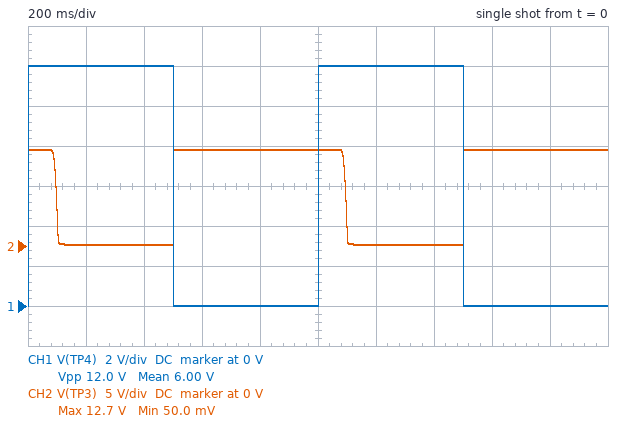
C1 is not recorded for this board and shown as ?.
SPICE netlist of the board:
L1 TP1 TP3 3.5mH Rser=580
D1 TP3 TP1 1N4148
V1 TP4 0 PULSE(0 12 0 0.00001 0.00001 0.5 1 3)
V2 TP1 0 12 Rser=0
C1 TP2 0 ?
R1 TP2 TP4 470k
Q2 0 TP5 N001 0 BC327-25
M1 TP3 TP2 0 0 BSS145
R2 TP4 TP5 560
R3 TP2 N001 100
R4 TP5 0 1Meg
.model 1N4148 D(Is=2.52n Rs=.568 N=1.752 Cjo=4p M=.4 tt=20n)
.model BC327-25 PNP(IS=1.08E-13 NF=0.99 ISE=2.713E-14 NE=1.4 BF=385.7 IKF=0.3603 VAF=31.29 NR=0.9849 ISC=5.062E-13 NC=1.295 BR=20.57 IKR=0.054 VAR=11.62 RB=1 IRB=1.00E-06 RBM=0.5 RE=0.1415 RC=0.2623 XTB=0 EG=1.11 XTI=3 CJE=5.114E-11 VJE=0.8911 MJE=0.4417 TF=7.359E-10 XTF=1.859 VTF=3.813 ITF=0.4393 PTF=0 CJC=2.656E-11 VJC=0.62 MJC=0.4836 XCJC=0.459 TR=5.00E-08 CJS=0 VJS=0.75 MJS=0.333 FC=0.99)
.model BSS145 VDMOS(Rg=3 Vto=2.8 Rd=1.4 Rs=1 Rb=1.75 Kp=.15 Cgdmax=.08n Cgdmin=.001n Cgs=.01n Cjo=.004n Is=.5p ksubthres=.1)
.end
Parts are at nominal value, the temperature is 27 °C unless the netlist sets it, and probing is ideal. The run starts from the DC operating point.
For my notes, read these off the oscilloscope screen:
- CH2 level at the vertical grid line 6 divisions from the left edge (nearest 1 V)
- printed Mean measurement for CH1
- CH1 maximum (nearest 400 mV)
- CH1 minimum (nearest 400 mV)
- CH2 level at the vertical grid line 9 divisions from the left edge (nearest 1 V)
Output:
0 V
6.00 V
12.0 V
0 V
12 V
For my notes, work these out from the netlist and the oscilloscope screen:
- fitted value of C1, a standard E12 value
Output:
680 nF
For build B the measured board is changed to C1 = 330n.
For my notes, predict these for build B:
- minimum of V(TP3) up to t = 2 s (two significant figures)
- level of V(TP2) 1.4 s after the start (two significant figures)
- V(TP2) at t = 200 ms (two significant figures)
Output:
65 mV
11 V
8.7 V
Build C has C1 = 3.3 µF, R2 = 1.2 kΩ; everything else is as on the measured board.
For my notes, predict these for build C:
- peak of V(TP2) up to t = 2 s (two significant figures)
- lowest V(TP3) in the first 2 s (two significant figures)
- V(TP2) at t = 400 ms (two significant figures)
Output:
3.5 V
280 mV
2.7 V
